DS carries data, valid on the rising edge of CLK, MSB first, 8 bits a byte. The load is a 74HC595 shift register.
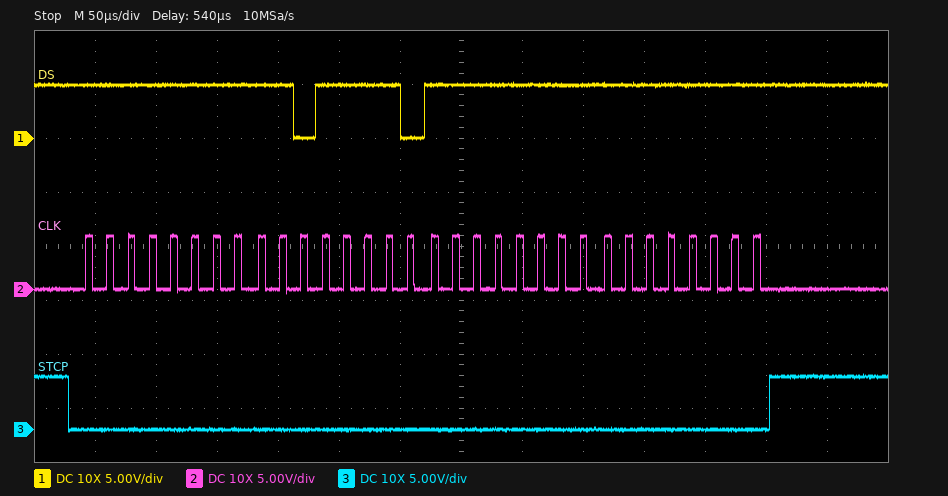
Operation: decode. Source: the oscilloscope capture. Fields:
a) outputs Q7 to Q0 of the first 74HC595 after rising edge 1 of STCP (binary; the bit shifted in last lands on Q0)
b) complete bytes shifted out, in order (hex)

11111111
0xFF 0xDE 0xFF 0xFF
